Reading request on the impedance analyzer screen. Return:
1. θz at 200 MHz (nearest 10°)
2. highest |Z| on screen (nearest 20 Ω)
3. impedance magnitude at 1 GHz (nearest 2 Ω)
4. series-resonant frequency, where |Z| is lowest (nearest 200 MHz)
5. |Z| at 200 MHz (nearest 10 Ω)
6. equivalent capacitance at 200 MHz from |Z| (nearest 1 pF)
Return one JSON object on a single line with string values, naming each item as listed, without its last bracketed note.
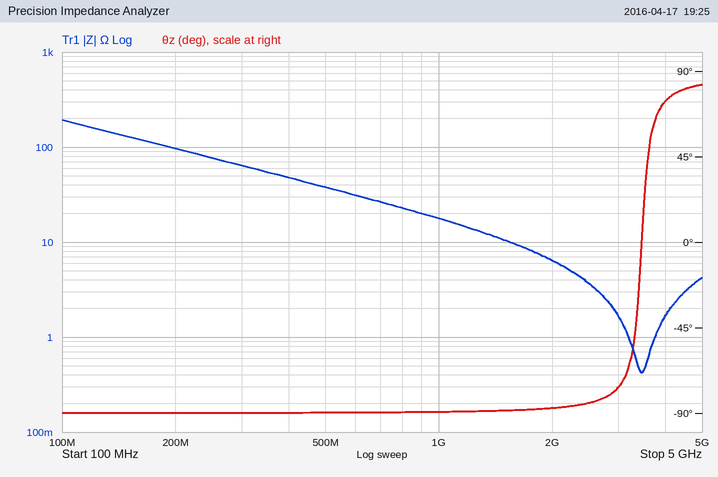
{"θz at 200 MHz": "-90°", "highest |Z| on screen": "200 Ω", "impedance magnitude at 1 GHz": "18 Ω", "series-resonant frequency, where |Z| is lowest": "3.4 GHz", "|Z| at 200 MHz": "100 Ω", "equivalent capacitance at 200 MHz from |Z|": "8 pF"}
